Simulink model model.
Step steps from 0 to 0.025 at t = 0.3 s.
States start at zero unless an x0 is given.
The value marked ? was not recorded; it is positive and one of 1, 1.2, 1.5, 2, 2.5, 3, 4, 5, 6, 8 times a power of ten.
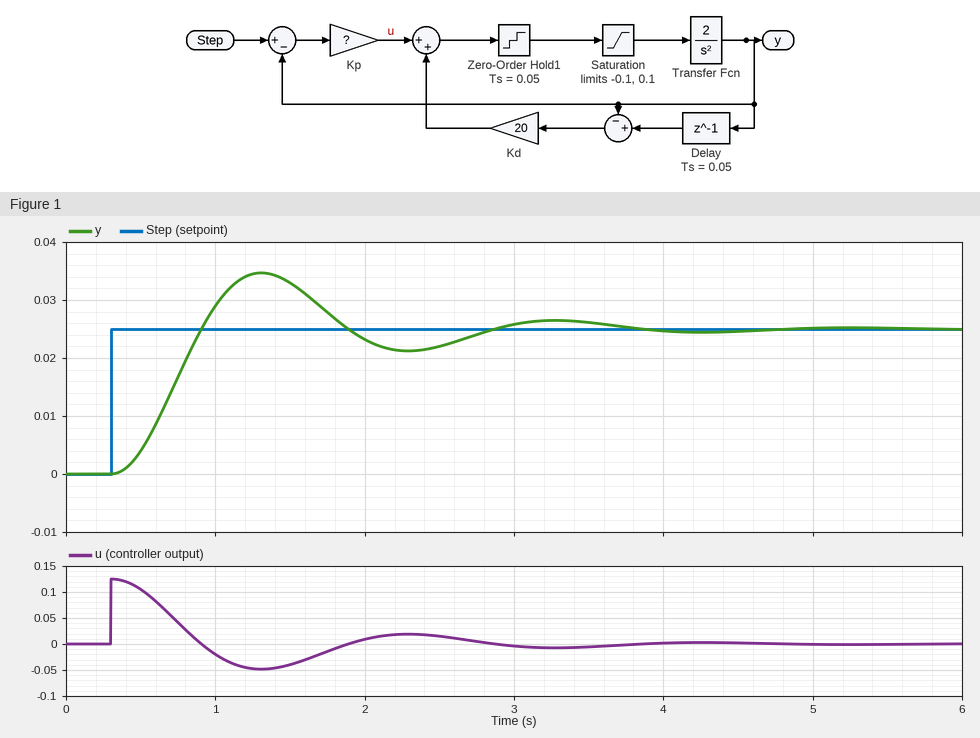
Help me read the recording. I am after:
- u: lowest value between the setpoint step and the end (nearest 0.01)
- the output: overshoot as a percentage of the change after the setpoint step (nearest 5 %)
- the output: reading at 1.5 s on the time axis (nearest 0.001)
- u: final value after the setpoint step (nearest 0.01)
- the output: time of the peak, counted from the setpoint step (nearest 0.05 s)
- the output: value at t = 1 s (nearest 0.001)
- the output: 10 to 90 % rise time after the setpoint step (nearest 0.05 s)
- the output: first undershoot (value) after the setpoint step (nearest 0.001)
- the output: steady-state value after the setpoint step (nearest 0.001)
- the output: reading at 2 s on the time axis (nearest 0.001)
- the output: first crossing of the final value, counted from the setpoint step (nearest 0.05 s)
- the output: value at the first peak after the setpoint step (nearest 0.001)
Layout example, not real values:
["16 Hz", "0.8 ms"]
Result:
["-0.05", "40 %", "0.033", "0.00", "1.00 s", "0.029", "0.40 s", "0.021", "0.025", "0.023", "0.60 s", "0.035"]
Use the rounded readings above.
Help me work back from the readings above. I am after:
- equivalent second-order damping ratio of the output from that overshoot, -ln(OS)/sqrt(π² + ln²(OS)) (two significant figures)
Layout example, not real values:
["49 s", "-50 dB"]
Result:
["0.28"]
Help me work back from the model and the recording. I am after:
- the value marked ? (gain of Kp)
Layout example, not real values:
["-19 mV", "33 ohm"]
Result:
["5"]
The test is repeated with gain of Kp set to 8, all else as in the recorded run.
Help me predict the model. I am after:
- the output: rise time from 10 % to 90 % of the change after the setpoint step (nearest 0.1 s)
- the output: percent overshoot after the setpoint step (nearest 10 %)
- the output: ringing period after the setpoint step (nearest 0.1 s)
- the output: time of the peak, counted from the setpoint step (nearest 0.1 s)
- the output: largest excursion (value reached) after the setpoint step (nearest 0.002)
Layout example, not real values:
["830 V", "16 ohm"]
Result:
["0.3 s", "50 %", "1.5 s", "0.9 s", "0.038"]
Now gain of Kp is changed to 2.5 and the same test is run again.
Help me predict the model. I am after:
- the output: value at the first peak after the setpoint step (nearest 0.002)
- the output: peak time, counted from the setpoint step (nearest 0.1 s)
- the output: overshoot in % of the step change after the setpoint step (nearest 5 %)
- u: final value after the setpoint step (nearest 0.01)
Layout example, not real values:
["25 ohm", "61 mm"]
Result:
["0.030", "1.5 s", "20 %", "0.00"]
